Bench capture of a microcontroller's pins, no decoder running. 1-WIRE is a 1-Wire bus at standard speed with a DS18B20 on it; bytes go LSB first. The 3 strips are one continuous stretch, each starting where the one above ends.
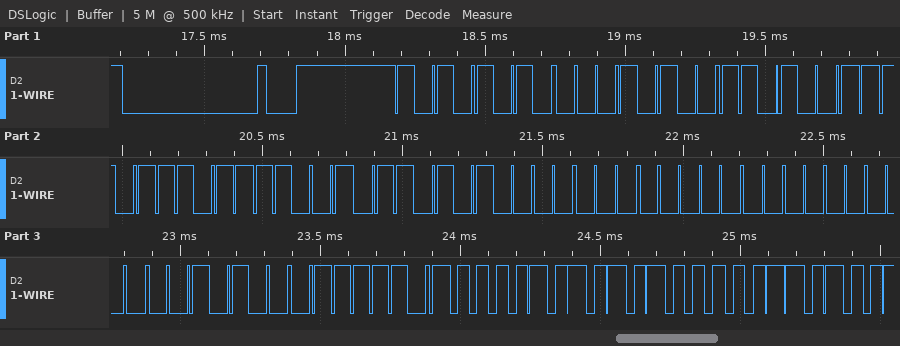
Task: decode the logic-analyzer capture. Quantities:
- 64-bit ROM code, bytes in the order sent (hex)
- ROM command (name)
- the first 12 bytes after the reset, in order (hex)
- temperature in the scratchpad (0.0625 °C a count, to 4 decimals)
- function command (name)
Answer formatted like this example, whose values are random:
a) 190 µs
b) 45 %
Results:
a) 28 CB DD D3 0A 00 00 28
b) Match ROM
c) 55 28 CB DD D3 0A 00 00 28 BE 50 05
d) 85.0000 °C
e) Read Scratchpad
